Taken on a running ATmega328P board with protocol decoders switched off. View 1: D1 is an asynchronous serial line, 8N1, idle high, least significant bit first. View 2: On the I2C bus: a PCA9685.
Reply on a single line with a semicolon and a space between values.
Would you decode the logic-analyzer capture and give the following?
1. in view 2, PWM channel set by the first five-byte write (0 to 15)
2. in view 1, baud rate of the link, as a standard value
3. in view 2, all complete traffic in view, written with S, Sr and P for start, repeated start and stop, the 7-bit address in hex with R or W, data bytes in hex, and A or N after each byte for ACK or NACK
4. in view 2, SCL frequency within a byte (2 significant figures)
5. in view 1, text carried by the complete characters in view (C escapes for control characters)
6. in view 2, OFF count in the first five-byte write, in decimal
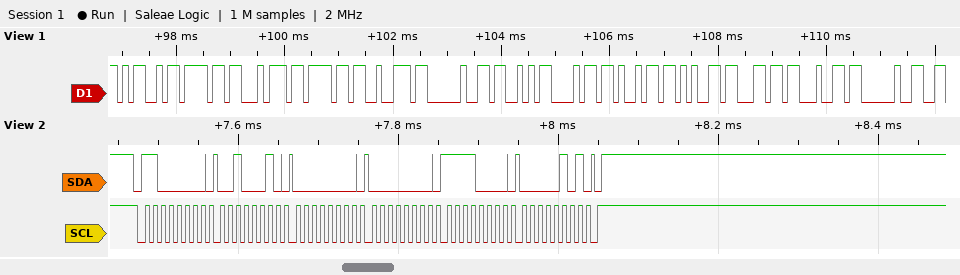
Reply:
7; 9600 baud; S 60W A 22 A 00 A 00 A F0 A 05 A P; 100 kHz; "Motor Shield "; 1520
